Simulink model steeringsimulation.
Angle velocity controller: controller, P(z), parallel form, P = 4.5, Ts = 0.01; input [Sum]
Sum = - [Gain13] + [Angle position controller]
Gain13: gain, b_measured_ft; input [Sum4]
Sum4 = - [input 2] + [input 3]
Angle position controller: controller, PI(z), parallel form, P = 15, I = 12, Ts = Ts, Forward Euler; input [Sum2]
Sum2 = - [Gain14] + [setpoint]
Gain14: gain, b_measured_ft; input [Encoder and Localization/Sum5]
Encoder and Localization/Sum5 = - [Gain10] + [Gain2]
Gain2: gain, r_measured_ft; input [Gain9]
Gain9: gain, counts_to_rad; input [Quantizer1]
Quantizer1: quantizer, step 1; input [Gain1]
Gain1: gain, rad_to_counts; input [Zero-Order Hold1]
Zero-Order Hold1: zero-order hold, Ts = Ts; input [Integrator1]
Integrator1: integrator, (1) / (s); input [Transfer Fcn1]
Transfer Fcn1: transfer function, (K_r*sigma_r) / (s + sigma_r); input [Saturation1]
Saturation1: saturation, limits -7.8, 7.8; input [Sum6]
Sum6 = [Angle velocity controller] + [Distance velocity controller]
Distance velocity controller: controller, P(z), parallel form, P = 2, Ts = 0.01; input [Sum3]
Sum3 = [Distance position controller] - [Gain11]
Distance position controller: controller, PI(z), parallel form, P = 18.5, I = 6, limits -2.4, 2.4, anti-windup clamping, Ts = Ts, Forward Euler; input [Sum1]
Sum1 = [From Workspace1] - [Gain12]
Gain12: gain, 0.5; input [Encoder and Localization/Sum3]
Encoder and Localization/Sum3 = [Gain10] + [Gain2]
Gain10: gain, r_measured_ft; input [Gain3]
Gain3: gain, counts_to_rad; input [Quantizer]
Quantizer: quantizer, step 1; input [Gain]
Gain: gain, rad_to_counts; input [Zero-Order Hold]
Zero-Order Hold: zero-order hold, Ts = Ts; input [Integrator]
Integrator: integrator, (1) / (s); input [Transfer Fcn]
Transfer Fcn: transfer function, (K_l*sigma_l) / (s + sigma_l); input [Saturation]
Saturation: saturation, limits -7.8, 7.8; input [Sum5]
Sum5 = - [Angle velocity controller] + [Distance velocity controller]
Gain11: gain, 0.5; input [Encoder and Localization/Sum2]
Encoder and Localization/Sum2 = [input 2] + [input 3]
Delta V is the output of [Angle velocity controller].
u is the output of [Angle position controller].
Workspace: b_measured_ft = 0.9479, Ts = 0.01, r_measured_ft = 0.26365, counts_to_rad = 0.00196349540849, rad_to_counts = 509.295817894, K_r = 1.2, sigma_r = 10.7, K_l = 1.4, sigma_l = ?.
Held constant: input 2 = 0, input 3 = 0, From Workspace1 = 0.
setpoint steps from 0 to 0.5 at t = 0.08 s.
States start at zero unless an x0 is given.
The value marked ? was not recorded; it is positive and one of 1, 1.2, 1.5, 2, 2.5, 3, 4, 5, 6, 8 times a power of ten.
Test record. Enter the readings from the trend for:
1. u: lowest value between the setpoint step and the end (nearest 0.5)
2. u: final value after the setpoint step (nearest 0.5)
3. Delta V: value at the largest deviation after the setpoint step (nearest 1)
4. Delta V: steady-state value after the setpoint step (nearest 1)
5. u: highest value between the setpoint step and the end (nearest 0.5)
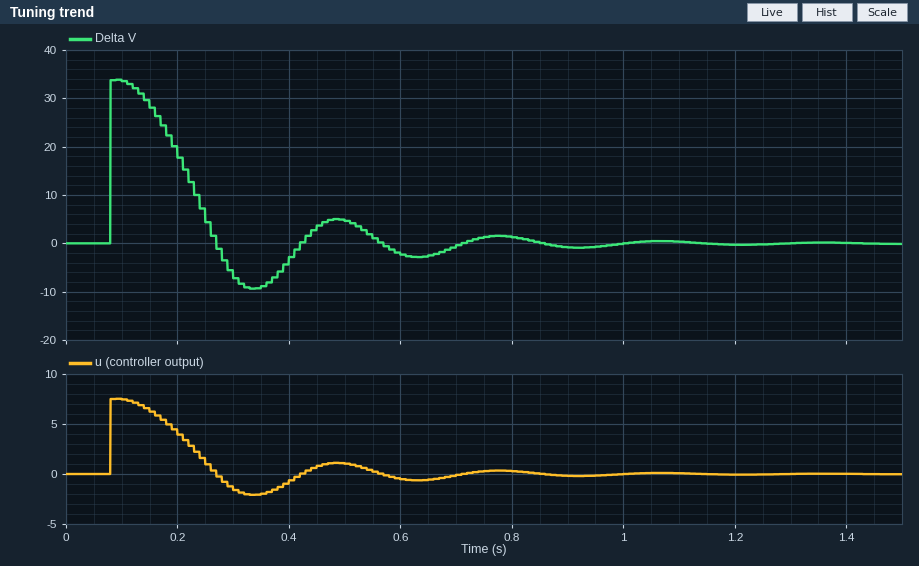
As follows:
-2.0
0.0
34
0
7.5
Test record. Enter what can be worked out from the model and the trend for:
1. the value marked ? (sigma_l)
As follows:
12
